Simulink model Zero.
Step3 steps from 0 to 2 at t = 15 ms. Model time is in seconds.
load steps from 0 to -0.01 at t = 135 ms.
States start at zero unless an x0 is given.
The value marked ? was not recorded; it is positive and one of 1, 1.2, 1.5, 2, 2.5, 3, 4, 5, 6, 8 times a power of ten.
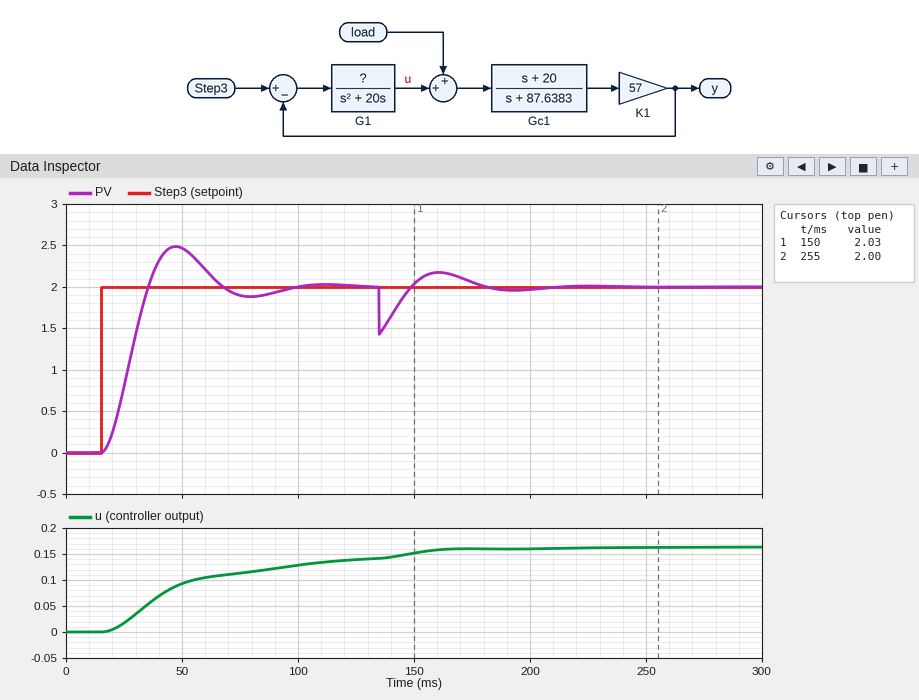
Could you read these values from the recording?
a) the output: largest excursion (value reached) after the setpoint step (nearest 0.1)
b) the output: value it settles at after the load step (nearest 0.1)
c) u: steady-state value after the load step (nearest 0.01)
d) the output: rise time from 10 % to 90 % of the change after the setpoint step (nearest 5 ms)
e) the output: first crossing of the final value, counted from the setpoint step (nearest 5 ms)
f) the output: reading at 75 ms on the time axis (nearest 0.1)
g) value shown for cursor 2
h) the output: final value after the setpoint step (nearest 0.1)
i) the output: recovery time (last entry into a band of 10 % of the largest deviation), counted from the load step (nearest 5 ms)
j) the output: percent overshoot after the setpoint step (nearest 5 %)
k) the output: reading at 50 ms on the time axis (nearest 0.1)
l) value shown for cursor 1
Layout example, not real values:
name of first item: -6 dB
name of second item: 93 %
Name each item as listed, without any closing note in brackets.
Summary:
the output: largest excursion (value reached) after the setpoint step: 2.5
the output: value it settles at after the load step: 2.0
u: steady-state value after the load step: 0.16
the output: rise time from 10 % to 90 % of the change after the setpoint step: 15 ms
the output: first crossing of the final value, counted from the setpoint step: 20 ms
the output: reading at 75 ms on the time axis: 1.9
value shown for cursor 2: 2.00
the output: final value after the setpoint step: 2.0
the output: recovery time (last entry into a band of 10 % of the largest deviation), counted from the load step: 40 ms
the output: percent overshoot after the setpoint step: 25 %
the output: reading at 50 ms on the time axis: 2.5
value shown for cursor 1: 2.03
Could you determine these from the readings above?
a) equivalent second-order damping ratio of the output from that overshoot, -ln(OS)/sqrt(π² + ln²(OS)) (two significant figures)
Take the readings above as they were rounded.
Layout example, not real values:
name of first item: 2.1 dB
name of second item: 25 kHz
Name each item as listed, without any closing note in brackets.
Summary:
equivalent second-order damping ratio of the output from that overshoot, -ln(OS)/sqrt(π² + ln²(OS)): 0.40
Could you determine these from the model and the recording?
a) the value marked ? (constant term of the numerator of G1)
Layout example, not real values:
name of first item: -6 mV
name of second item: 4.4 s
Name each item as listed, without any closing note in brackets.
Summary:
the value marked ?: 200
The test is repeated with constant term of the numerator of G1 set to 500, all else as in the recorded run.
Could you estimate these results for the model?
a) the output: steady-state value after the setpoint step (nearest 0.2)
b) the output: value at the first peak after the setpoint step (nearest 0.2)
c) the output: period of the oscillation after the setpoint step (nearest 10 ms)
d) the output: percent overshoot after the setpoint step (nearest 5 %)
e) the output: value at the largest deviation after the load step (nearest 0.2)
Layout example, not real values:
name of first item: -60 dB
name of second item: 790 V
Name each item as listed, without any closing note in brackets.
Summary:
the output: steady-state value after the setpoint step: 2.0
the output: value at the first peak after the setpoint step: 2.8
the output: period of the oscillation after the setpoint step: 40 ms
the output: percent overshoot after the setpoint step: 45 %
the output: value at the largest deviation after the load step: 1.4
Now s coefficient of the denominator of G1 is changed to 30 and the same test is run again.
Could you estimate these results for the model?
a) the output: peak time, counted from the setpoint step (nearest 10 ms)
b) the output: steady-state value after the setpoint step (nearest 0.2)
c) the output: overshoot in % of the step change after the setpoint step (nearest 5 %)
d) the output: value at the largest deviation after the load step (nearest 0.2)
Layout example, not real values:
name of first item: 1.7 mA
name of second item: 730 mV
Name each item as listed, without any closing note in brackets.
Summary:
the output: peak time, counted from the setpoint step: 30 ms
the output: steady-state value after the setpoint step: 2.0
the output: overshoot in % of the step change after the setpoint step: 15 %
the output: value at the largest deviation after the load step: 1.4
